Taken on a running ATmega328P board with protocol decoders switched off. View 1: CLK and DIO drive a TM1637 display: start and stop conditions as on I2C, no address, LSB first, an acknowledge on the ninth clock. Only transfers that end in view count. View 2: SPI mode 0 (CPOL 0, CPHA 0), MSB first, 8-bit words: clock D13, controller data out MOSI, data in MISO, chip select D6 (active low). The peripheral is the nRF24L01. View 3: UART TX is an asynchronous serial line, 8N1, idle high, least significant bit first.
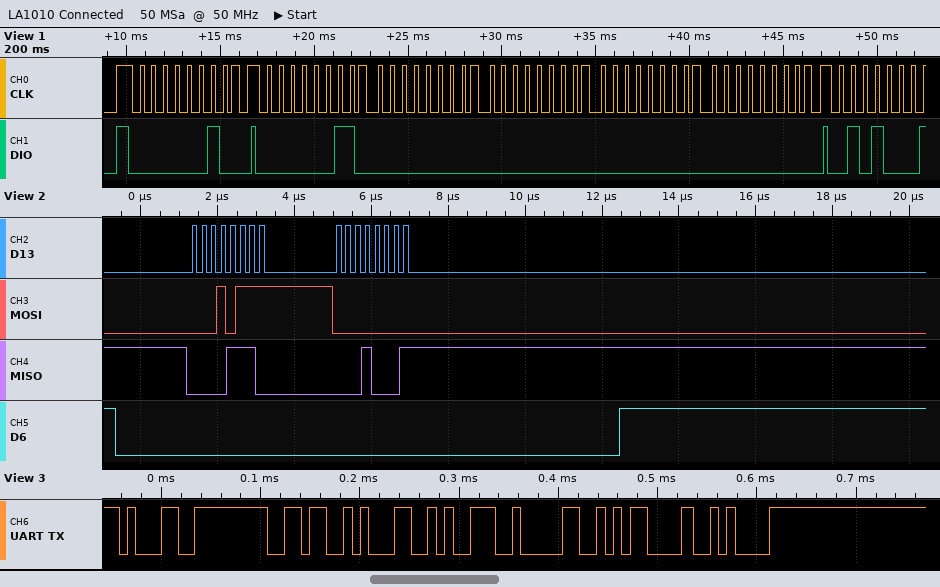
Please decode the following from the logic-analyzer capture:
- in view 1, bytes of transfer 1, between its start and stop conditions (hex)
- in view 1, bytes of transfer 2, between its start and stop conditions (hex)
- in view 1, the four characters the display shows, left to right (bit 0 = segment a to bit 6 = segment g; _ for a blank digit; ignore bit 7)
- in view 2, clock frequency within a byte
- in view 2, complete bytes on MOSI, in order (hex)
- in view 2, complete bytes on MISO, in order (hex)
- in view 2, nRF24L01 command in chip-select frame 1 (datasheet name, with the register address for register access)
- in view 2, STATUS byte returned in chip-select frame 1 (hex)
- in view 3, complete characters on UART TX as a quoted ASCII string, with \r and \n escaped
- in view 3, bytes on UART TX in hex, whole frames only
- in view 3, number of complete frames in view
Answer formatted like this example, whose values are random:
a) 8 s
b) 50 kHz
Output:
a) 40
b) C0 00 00 00 00
c) ____
d) 4 MHz
e) 17 00
f) 0E 11
g) R_REGISTER 0x17
h) 0x0E
i) "16190\r\n"
j) 31 36 31 39 30 0D 0A
k) 7
